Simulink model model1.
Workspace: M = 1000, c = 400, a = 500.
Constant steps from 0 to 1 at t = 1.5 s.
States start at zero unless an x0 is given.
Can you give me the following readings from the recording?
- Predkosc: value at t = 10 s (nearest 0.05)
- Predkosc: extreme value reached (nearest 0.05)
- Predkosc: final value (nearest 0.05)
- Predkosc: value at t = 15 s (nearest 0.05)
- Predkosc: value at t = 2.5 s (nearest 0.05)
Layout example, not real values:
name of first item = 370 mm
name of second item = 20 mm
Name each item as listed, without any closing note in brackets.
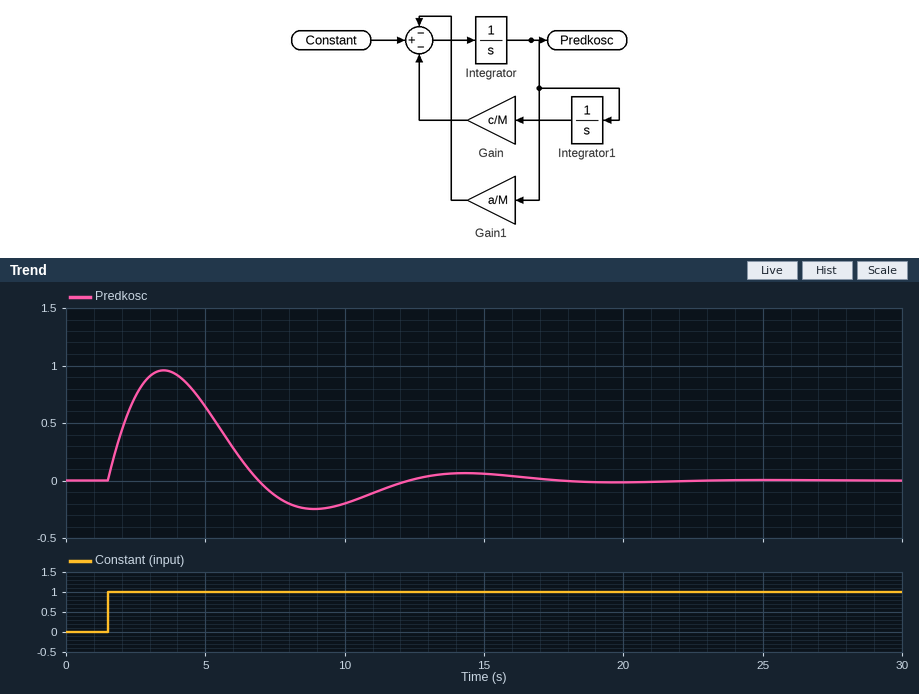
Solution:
Predkosc: value at t = 10 s = -0.20
Predkosc: extreme value reached = 0.95
Predkosc: final value = 0.00
Predkosc: value at t = 15 s = 0.05
Predkosc: value at t = 2.5 s = 0.75
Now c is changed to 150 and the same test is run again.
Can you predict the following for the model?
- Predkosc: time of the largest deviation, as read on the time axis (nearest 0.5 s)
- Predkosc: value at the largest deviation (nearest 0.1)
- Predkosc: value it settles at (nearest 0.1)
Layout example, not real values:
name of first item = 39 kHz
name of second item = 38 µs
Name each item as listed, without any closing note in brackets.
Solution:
Predkosc: time of the largest deviation, as read on the time axis = 4.5 s
Predkosc: value at the largest deviation = 1.2
Predkosc: value it settles at = 0.0
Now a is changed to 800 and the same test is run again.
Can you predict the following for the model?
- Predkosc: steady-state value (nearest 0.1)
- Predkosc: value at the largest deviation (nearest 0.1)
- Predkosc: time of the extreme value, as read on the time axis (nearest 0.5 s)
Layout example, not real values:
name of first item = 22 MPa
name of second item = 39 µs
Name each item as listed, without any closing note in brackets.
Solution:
Predkosc: steady-state value = 0.0
Predkosc: value at the largest deviation = 0.8
Predkosc: time of the extreme value, as read on the time axis = 3.5 s
